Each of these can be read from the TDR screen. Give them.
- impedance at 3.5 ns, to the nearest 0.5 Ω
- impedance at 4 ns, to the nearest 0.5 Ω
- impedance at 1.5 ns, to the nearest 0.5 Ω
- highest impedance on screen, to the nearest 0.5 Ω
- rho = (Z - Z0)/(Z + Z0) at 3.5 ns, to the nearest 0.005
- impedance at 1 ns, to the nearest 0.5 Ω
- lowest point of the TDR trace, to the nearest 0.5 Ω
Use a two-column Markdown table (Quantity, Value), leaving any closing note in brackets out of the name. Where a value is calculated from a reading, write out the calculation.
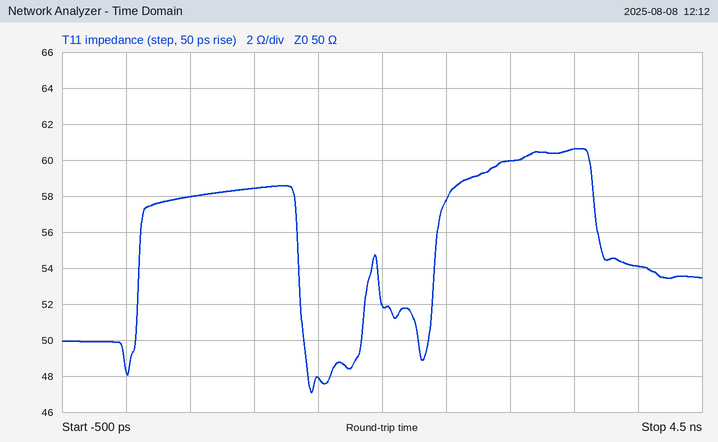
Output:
| Quantity | Value |
|---|---|
| impedance at 3.5 ns, to the nearest 0.5 Ω | 60.5 Ω |
| impedance at 4 ns, to the nearest 0.5 Ω | 54.0 Ω |
| impedance at 1.5 ns, to the nearest 0.5 Ω | 48.0 Ω |
| highest impedance on screen, to the nearest 0.5 Ω | 60.5 Ω |
| rho = (Z - Z0)/(Z + Z0) at 3.5 ns, to the nearest 0.005 | (60.5 − 50)/(60.5 + 50) ≈ +0.095 |
| impedance at 1 ns, to the nearest 0.5 Ω | 58.5 Ω |
| lowest point of the TDR trace, to the nearest 0.5 Ω | 47.0 Ω |
